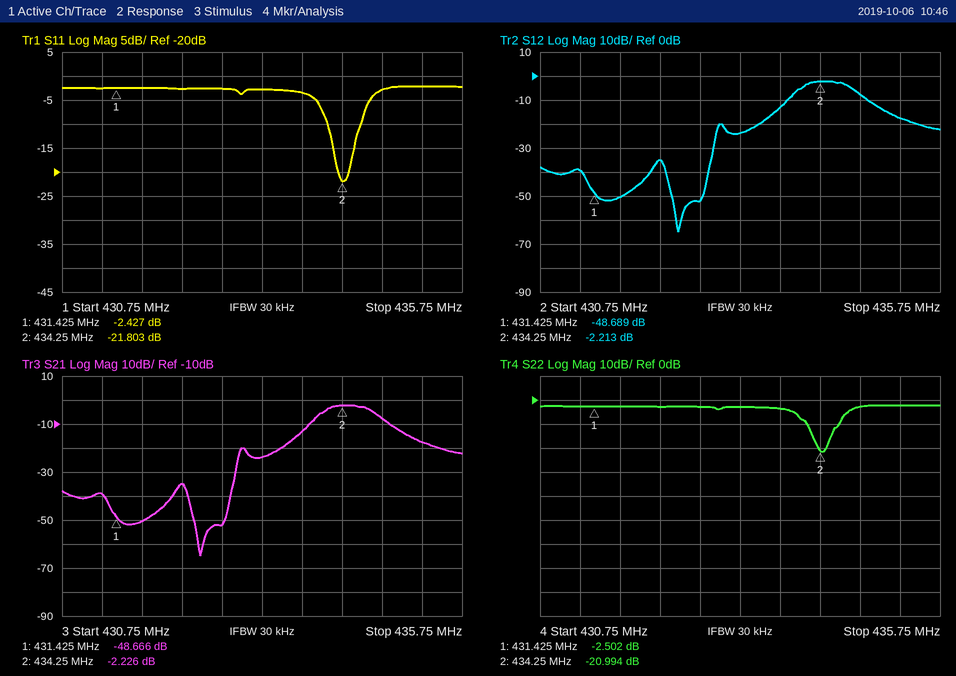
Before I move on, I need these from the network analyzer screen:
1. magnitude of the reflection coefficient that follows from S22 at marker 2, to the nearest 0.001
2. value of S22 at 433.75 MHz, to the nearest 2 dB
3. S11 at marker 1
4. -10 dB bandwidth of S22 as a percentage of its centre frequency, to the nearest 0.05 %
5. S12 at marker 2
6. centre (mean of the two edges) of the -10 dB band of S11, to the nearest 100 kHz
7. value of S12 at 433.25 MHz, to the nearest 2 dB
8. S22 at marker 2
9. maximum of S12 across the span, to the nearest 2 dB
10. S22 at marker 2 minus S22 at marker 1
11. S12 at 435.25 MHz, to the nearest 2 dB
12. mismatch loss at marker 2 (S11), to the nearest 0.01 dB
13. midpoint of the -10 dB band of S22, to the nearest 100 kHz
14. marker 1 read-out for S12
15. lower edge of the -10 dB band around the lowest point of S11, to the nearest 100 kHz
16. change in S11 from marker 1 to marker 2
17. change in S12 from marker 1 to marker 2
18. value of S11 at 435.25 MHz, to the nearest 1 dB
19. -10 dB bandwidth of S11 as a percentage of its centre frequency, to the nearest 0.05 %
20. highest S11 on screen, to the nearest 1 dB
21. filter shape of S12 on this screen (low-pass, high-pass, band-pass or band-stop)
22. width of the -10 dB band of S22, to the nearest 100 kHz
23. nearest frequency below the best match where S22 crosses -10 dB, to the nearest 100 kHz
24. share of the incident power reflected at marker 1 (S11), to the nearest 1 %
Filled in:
0.089
-4 dB
-2.427 dB
0.10 %
-2.213 dB
434.3 MHz
-24 dB
-20.994 dB
-2 dB
-18.492 dB
-18 dB
0.03 dB
434.3 MHz
-48.689 dB
434.1 MHz
-19.376 dB
46.476 dB
-2 dB
0.10 %
-2 dB
band-pass
400 kHz
434.1 MHz
57 %
